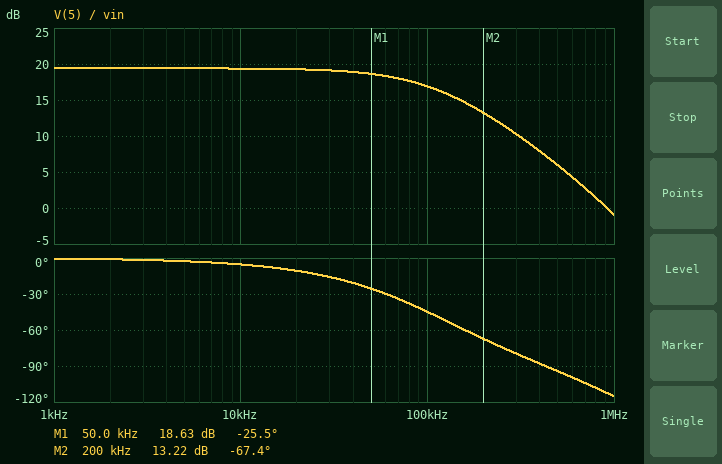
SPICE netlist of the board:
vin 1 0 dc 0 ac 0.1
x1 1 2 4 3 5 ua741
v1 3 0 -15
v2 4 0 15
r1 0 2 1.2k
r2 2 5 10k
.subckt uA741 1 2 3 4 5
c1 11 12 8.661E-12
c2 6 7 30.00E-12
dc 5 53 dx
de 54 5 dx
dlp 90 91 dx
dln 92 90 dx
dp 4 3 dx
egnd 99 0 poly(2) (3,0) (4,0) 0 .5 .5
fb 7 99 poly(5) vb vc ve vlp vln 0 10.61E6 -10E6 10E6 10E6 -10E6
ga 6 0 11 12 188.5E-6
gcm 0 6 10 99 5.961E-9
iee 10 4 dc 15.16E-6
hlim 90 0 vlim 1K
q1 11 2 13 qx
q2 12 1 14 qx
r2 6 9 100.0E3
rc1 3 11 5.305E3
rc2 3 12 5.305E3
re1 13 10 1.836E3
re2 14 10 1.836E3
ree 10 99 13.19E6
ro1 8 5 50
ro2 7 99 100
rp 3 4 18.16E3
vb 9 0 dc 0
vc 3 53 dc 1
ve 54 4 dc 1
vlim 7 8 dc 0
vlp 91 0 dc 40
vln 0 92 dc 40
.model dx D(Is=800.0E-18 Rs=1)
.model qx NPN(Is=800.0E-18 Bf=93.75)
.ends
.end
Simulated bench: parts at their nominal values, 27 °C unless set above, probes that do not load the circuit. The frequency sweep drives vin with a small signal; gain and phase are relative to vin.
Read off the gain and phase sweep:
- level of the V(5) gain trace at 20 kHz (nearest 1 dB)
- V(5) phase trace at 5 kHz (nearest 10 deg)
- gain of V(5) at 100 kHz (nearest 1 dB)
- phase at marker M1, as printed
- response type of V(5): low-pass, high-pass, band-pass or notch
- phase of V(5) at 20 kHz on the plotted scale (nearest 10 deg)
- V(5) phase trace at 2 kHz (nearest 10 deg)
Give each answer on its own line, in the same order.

19 dB
0 deg
17 dB
-25.5 deg
low-pass
-10 deg
0 deg
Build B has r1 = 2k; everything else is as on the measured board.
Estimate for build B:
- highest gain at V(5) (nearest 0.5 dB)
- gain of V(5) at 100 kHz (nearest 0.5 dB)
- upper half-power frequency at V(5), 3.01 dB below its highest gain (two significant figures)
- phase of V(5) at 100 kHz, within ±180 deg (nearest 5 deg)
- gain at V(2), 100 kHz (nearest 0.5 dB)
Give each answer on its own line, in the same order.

15.5 dB
14.5 dB
180 kHz
-30 deg
-1.0 dB
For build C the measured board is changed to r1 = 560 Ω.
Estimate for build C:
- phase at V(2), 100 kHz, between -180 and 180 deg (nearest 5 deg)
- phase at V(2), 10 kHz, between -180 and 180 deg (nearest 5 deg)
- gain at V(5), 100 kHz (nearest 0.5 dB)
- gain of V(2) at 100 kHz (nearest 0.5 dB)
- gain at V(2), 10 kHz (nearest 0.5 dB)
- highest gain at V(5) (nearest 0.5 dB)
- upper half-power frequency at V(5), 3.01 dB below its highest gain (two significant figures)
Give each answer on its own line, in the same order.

-65 deg
-10 deg
19.0 dB
-6.5 dB
0 dB
25.5 dB
54 kHz
